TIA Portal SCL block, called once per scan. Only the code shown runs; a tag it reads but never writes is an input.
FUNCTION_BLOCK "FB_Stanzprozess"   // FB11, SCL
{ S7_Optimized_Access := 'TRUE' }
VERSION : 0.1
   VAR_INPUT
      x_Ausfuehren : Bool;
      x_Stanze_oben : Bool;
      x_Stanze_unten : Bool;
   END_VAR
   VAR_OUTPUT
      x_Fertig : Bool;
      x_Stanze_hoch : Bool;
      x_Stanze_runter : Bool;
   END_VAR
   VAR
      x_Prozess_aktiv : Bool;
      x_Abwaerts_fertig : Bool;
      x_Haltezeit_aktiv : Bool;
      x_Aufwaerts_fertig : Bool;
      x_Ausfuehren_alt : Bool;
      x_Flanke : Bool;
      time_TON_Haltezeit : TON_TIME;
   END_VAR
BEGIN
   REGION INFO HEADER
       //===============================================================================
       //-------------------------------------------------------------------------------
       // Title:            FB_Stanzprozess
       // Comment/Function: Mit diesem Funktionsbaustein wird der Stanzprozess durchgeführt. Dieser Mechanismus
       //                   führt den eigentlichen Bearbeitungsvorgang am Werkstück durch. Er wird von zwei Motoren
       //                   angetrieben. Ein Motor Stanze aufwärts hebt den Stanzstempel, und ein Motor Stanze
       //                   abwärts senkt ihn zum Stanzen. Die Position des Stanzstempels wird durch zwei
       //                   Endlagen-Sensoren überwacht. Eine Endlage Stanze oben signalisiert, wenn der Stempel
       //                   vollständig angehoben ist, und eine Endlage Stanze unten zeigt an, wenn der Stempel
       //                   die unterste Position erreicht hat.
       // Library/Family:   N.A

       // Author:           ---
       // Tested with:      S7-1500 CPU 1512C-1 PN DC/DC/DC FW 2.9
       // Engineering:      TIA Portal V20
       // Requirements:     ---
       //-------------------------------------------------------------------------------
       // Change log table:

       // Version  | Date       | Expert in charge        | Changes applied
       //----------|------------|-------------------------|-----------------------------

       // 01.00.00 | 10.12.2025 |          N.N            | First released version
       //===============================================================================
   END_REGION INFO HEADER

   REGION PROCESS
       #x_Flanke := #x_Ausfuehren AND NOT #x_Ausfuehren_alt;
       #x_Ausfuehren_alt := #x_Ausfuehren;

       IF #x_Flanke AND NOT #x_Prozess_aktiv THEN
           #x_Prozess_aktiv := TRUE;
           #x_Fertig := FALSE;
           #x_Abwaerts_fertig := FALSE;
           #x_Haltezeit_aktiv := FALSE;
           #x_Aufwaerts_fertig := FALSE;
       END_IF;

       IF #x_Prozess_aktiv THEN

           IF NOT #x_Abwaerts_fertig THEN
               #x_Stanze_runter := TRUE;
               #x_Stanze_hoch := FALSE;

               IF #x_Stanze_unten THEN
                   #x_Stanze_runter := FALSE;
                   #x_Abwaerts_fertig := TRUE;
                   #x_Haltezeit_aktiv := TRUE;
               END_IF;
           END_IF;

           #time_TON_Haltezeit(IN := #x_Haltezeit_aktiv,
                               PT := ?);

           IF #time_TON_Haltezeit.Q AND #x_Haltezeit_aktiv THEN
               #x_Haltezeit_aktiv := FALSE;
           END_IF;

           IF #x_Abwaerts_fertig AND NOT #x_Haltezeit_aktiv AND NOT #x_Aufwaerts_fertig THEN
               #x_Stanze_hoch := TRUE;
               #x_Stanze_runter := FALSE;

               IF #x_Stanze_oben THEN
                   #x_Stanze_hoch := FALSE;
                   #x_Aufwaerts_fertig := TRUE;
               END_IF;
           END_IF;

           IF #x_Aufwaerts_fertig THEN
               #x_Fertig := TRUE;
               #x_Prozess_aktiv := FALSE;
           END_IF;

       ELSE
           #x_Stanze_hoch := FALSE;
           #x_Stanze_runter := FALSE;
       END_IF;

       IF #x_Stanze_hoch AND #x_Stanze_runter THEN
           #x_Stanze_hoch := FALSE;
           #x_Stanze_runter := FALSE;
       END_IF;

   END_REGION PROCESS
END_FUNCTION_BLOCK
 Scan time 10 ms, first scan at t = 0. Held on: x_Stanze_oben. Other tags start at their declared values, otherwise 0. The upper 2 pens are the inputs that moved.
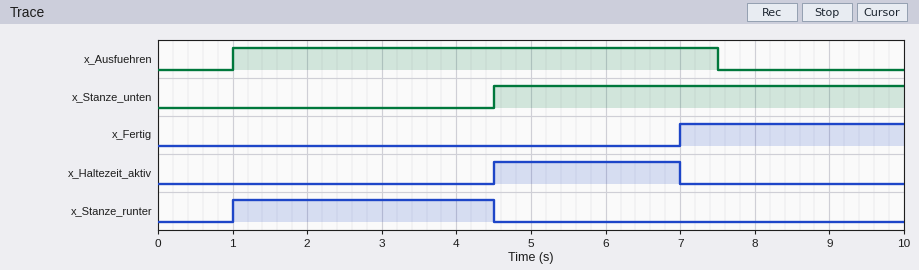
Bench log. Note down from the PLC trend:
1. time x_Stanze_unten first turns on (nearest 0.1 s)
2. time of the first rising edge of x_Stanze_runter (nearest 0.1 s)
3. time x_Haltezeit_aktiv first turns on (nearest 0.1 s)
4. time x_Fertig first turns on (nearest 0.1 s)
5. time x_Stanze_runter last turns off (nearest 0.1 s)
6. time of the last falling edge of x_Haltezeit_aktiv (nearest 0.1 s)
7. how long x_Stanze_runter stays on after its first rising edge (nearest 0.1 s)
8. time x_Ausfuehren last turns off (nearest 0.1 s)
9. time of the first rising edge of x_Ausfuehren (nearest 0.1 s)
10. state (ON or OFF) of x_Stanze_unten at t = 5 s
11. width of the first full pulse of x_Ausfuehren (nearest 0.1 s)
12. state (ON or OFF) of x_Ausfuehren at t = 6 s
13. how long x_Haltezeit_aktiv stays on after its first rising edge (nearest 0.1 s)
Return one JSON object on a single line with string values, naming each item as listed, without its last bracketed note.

{"time x_Stanze_unten first turns on": "4.5 s", "time of the first rising edge of x_Stanze_runter": "1.0 s", "time x_Haltezeit_aktiv first turns on": "4.5 s", "time x_Fertig first turns on": "7.0 s", "time x_Stanze_runter last turns off": "4.5 s", "time of the last falling edge of x_Haltezeit_aktiv": "7.0 s", "how long x_Stanze_runter stays on after its first rising edge": "3.5 s", "time x_Ausfuehren last turns off": "7.5 s", "time of the first rising edge of x_Ausfuehren": "1.0 s", "state (ON or OFF) of x_Stanze_unten at t = 5 s": "ON", "width of the first full pulse of x_Ausfuehren": "6.5 s", "state (ON or OFF) of x_Ausfuehren at t = 6 s": "ON", "how long x_Haltezeit_aktiv stays on after its first rising edge": "2.5 s"}
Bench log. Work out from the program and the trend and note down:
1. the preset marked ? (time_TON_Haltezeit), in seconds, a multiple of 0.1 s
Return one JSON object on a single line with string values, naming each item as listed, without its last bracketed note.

{"the preset marked ? (time_TON_Haltezeit), in seconds, a multiple of 0.1 s": "2.5 s"}
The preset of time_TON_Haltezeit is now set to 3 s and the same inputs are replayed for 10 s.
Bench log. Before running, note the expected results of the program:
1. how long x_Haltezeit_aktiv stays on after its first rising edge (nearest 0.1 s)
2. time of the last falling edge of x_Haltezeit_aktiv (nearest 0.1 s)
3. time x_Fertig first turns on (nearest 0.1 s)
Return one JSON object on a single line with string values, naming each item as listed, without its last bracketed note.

{"how long x_Haltezeit_aktiv stays on after its first rising edge": "3.0 s", "time of the last falling edge of x_Haltezeit_aktiv": "7.5 s", "time x_Fertig first turns on": "7.5 s"}
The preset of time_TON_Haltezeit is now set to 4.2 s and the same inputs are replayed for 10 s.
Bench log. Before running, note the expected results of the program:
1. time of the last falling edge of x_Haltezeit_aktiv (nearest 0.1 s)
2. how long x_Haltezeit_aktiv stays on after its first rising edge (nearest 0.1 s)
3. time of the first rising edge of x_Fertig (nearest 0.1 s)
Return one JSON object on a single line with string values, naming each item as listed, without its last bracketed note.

{"time of the last falling edge of x_Haltezeit_aktiv": "8.7 s", "how long x_Haltezeit_aktiv stays on after its first rising edge": "4.2 s", "time of the first rising edge of x_Fertig": "8.7 s"}
